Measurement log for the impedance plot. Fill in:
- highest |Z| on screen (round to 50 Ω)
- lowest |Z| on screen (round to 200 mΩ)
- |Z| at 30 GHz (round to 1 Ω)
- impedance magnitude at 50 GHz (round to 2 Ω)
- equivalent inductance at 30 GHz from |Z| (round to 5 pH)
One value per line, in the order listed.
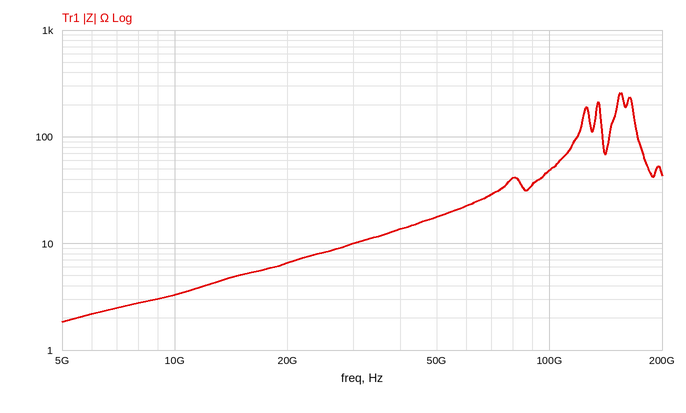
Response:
250 Ω
1.8 Ω
10 Ω
18 Ω
55 pH
